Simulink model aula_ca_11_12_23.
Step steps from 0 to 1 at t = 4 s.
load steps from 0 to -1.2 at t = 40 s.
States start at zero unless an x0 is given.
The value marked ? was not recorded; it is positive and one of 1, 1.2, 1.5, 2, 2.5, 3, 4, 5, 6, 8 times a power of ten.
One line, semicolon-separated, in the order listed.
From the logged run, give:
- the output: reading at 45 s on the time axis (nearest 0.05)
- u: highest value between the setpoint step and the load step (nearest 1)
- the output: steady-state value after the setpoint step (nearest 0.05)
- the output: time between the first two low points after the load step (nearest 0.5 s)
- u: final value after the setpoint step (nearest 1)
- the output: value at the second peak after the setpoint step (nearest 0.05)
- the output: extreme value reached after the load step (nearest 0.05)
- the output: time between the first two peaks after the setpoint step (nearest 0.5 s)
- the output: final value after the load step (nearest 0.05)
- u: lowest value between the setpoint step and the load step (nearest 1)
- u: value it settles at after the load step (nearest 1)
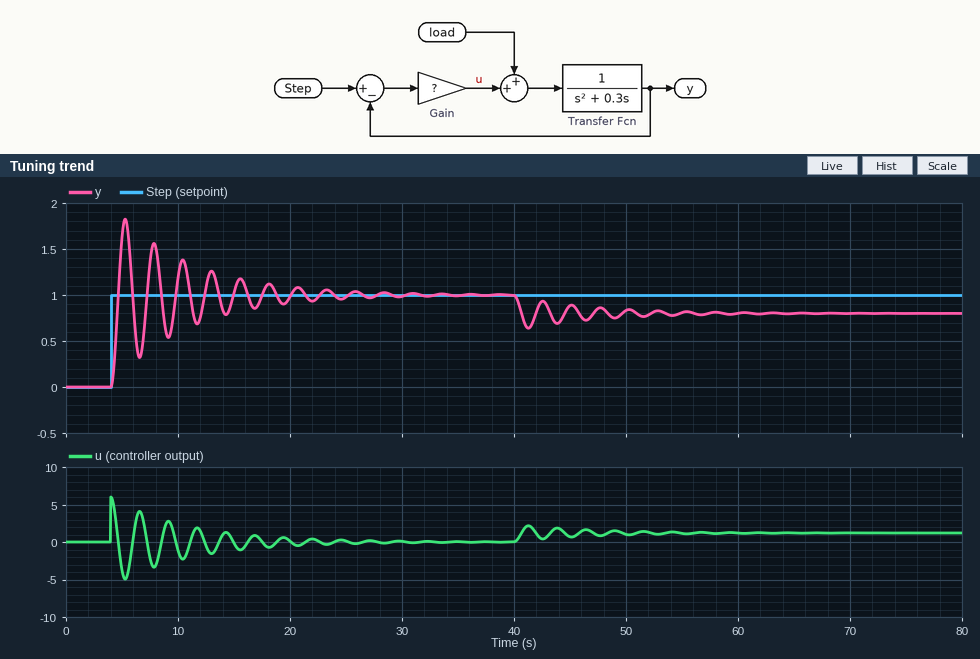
0.90; 6; 1.00; 2.5 s; 0; 1.55; 0.65; 2.5 s; 0.80; -5; 1
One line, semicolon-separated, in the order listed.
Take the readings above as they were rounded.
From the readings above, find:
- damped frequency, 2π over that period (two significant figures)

2.5 rad/s
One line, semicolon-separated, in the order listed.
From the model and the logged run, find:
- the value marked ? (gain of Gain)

6
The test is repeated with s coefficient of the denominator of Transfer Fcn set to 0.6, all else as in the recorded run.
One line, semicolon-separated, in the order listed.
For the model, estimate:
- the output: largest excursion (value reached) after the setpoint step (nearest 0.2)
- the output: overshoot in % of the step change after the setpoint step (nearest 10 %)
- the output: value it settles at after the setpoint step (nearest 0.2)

1.6; 70 %; 1.0
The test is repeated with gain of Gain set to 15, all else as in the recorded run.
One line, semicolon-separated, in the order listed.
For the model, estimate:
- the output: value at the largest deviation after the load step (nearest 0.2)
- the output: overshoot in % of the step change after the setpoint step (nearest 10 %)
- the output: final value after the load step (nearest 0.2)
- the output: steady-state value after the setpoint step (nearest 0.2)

0.8; 90 %; 1.0; 1.0
